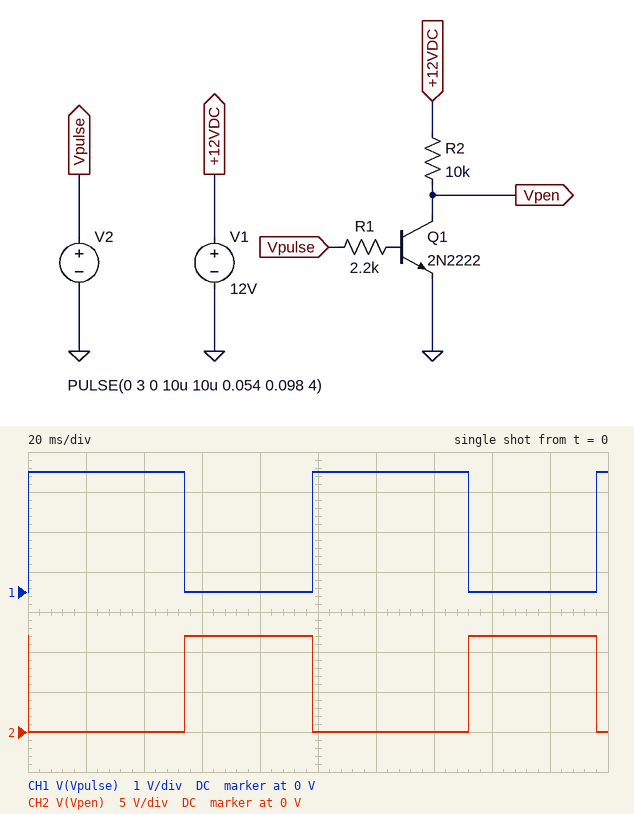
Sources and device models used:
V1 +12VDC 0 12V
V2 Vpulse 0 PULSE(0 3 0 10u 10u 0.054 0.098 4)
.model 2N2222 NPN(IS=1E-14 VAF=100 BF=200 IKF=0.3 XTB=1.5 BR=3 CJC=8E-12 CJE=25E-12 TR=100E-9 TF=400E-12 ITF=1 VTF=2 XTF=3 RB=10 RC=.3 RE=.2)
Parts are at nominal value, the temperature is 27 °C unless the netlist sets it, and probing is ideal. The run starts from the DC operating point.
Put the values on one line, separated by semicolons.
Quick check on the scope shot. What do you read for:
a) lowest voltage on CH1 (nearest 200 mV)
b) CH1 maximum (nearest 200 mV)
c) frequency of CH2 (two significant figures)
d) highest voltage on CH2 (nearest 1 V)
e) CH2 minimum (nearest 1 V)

0 V; 3.0 V; 10 Hz; 12 V; 0 V
